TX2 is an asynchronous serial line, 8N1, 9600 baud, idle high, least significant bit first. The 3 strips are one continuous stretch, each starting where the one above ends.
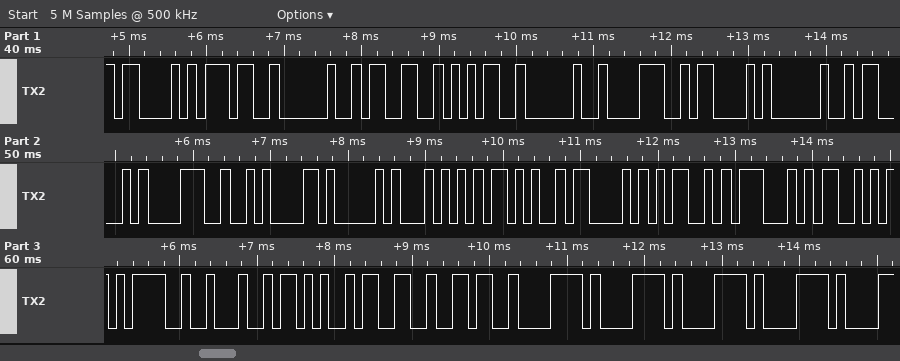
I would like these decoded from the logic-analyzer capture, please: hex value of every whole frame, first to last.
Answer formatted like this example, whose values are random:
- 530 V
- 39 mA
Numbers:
- 0x43 0x37 0x20 0x33 0x35 0x20 0x38 0x43 0x20 0x43 0x38 0x0A 0x41 0x54 0x2B 0x43 0x4D 0x47 0x53 0x3D 0x22 0x2B 0x33 0x36 0x78 0x78 0x78 0x78
